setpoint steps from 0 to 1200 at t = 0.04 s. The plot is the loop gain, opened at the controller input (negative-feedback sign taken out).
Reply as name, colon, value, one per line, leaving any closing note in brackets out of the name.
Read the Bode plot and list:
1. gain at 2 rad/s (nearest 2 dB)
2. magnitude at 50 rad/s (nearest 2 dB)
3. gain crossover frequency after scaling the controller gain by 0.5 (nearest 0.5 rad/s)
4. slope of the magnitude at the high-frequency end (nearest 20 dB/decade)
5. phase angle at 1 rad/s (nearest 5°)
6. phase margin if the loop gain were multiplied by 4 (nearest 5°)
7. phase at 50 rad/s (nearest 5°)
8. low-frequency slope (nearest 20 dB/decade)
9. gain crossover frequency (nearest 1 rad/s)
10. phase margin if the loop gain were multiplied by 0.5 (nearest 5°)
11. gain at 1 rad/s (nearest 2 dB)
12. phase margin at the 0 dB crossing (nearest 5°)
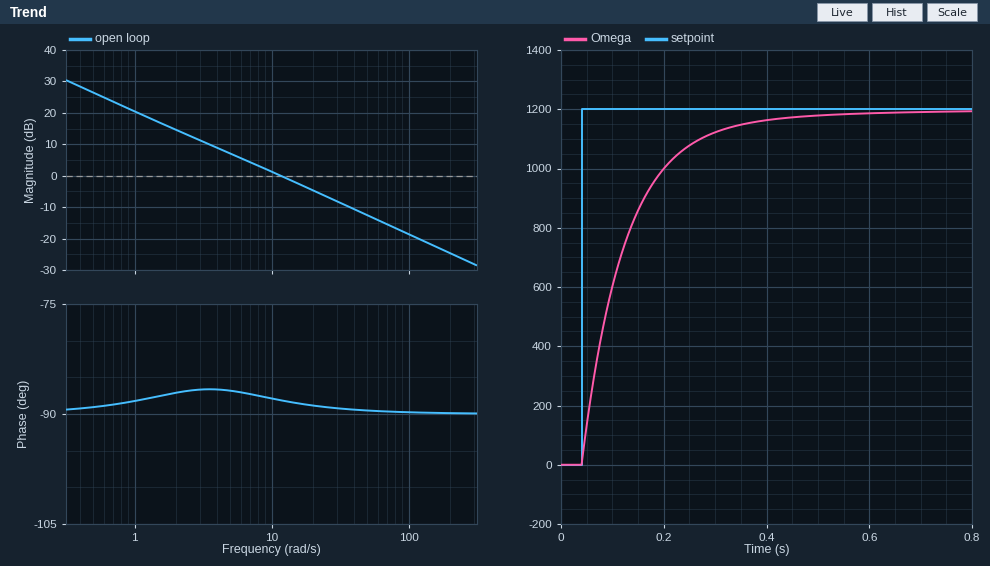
gain at 2 rad/s: 14 dB
magnitude at 50 rad/s: -12 dB
gain crossover frequency after scaling the controller gain by 0.5: 5.5 rad/s
slope of the magnitude at the high-frequency end: -20 dB/decade
phase angle at 1 rad/s: -90°
phase margin if the loop gain were multiplied by 4: 90°
phase at 50 rad/s: -90°
low-frequency slope: -20 dB/decade
gain crossover frequency: 12 rad/s
phase margin if the loop gain were multiplied by 0.5: 95°
gain at 1 rad/s: 20 dB
phase margin at the 0 dB crossing: 90°
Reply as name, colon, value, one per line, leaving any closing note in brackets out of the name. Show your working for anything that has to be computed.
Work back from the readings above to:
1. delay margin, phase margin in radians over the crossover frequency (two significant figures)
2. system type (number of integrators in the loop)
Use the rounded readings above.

delay margin, phase margin in radians over the crossover frequency: 90 × π / 180 / 12 = 0.13 s
system type: 1
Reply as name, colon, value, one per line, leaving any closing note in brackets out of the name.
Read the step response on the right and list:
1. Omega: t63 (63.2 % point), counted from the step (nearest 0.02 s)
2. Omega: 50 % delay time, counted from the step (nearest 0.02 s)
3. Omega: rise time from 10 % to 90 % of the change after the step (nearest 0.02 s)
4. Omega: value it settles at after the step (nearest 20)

Omega: t63 (63.2 % point), counted from the step: 0.08 s
Omega: 50 % delay time, counted from the step: 0.06 s
Omega: rise time from 10 % to 90 % of the change after the step: 0.20 s
Omega: value it settles at after the step: 1200
